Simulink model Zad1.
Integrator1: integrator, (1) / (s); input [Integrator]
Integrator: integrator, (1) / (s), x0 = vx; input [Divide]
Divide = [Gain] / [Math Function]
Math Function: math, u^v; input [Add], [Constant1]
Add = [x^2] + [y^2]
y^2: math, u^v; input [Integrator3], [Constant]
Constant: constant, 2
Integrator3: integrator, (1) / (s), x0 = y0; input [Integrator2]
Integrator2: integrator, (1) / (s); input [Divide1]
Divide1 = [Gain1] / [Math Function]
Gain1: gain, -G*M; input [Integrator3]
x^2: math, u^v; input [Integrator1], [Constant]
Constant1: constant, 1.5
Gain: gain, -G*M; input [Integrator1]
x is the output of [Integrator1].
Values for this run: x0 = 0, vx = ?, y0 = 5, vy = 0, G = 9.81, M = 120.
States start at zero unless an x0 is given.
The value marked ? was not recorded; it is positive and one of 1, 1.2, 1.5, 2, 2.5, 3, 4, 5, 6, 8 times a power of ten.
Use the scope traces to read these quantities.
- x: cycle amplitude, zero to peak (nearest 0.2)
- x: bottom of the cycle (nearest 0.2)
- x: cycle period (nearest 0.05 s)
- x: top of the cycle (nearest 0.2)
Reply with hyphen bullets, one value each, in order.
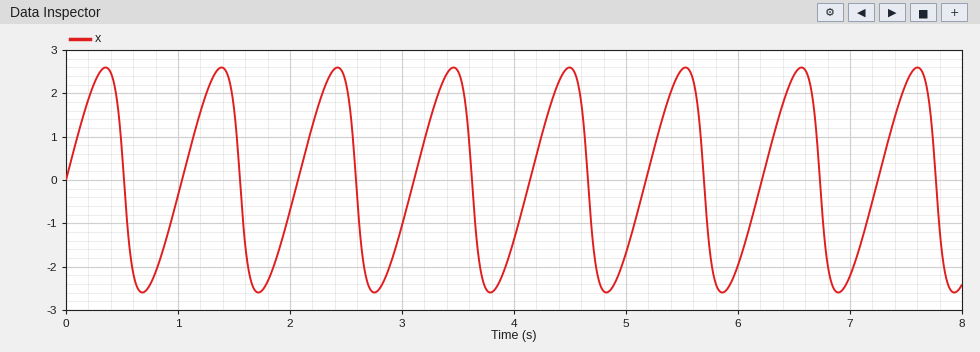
- 2.6
- -2.6
- 1.05 s
- 2.6
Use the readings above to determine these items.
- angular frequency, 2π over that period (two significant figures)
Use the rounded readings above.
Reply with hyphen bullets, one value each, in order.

- 6.0 rad/s
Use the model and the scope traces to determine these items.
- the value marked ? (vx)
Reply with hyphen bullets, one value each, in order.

- 10
